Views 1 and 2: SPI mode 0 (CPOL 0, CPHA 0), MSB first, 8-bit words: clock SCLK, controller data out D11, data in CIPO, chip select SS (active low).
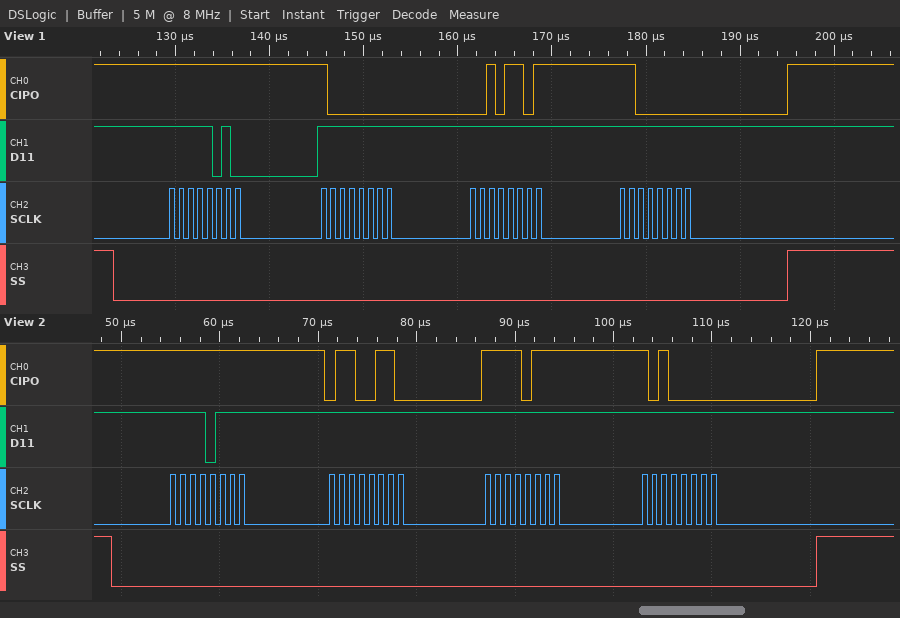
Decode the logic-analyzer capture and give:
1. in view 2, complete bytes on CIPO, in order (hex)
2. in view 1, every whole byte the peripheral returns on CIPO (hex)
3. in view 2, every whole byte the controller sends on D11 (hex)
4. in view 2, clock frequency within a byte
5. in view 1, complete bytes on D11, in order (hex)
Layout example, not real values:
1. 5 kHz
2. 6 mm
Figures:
1. FF 66 F7 A0
2. 0xFF 0x80 0x2D 0xC0
3. F7 FF FF FF
4. 1 MHz
5. 0xFA 0xFF 0xFF 0xFF
